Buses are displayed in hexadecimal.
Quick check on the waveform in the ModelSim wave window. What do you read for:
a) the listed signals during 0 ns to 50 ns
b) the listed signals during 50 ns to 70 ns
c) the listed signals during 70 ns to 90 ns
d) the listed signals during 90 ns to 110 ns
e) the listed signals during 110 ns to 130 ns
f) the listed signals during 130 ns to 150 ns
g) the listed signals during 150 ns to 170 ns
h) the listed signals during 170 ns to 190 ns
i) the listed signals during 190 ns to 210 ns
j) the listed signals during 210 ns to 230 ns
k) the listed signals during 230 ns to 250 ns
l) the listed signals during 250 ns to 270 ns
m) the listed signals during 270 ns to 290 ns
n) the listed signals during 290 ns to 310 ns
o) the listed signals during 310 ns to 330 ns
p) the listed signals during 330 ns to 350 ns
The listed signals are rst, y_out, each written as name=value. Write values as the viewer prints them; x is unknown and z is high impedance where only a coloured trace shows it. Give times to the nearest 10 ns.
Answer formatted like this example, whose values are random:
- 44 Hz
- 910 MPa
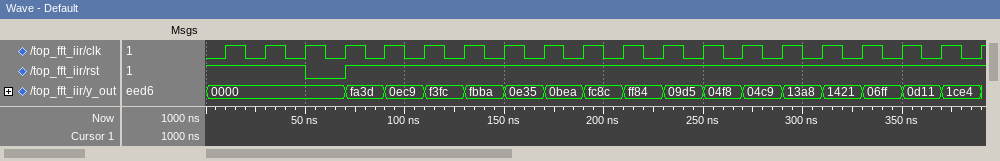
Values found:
- rst=1, y_out=0000
- rst=0, y_out=0000
- rst=1, y_out=fa3d
- rst=1, y_out=0ec9
- rst=1, y_out=f3fc
- rst=1, y_out=fbba
- rst=1, y_out=0e35
- rst=1, y_out=0bea
- rst=1, y_out=fc8c
- rst=1, y_out=ff84
- rst=1, y_out=09d5
- rst=1, y_out=04f8
- rst=1, y_out=04c9
- rst=1, y_out=13a8
- rst=1, y_out=1421
- rst=1, y_out=06ff
